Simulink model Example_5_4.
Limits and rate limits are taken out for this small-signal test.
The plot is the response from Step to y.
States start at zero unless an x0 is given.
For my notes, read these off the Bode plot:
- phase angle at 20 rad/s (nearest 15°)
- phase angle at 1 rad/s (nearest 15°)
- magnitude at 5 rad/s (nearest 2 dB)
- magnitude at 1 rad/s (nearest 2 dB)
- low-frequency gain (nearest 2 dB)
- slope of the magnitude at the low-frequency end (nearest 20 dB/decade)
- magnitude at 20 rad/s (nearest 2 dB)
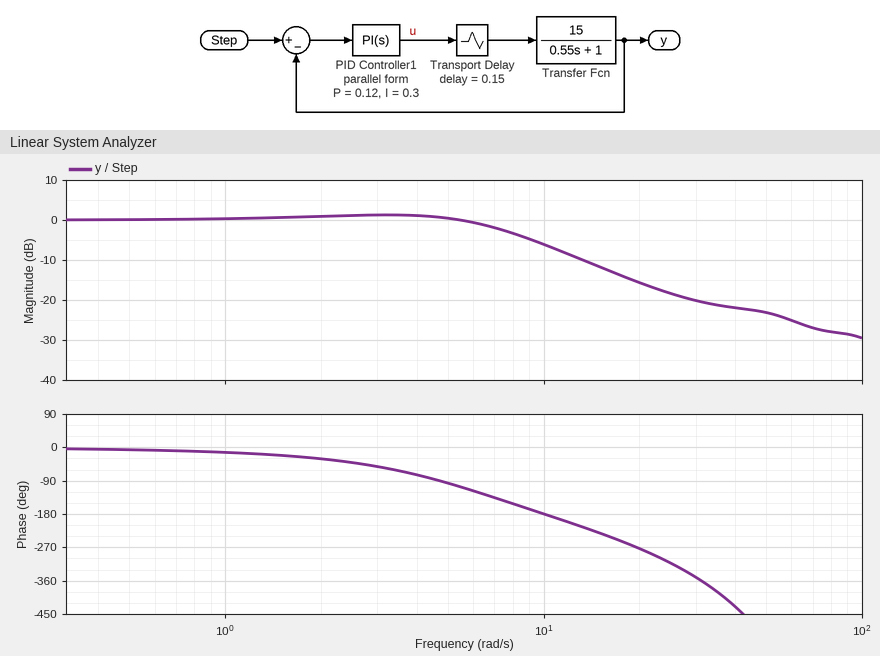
-270°
-15°
0 dB
0 dB
0 dB
0 dB/decade
-16 dB
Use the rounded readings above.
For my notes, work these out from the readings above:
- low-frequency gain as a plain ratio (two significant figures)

1.0
